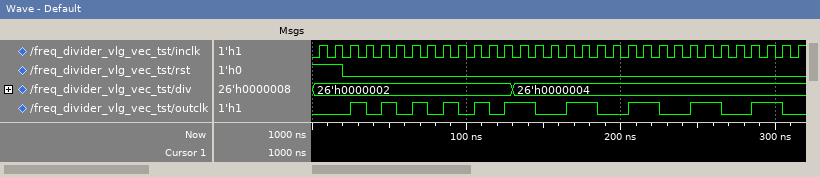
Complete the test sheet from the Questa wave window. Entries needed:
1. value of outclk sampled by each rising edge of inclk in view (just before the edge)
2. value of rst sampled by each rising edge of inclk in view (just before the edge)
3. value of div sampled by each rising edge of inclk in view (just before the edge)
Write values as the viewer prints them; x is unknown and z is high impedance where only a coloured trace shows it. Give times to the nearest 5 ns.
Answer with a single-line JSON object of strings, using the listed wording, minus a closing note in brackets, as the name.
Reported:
{"value of outclk sampled by each rising edge of inclk in view": "0 0 0 1 0 1 0 1 0 1 0 1 0 1 1 0 0 1 1 0 0 1 1 0 0 1 1 0 0 1 1 0", "value of rst sampled by each rising edge of inclk in view": "1 1 0 0 0 0 0 0 0 0 0 0 0 0 0 0 0 0 0 0 0 0 0 0 0 0 0 0 0 0 0 0", "value of div sampled by each rising edge of inclk in view": "26'h0000002, 26'h0000002, 26'h0000002, 26'h0000002, 26'h0000002, 26'h0000002, 26'h0000002, 26'h0000002, 26'h0000002, 26'h0000002, 26'h0000002, 26'h0000002, 26'h0000002, 26'h0000004, 26'h0000004, 26'h0000004, 26'h0000004, 26'h0000004, 26'h0000004, 26'h0000004, 26'h0000004, 26'h0000004, 26'h0000004, 26'h0000004, 26'h0000004, 26'h0000004, 26'h0000004, 26'h0000004, 26'h0000004, 26'h0000004, 26'h0000004, 26'h0000004"}
